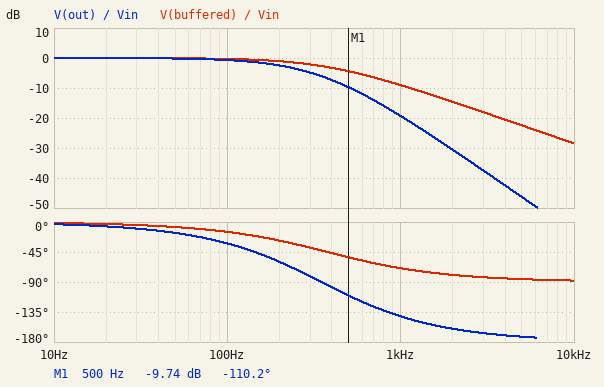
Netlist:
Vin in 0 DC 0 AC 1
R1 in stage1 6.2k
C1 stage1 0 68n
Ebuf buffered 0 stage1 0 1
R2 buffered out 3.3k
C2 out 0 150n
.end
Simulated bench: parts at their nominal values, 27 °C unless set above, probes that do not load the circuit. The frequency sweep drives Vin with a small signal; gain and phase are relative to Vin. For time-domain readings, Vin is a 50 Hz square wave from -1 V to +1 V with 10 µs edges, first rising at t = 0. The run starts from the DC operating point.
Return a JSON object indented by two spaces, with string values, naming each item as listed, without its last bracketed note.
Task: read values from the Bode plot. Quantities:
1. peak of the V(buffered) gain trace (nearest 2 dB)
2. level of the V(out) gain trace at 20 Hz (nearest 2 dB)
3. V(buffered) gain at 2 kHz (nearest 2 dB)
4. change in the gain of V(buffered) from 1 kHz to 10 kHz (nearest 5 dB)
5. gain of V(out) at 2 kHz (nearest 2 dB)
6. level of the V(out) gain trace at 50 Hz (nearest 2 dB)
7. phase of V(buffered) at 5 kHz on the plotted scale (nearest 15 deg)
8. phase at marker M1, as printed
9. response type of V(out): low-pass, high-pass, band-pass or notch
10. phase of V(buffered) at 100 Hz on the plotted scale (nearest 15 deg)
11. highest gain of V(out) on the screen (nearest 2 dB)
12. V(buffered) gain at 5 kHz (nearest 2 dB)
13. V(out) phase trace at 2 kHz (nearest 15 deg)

{
  "peak of the V(buffered) gain trace": "0 dB",
  "level of the V(out) gain trace at 20 Hz": "0 dB",
  "V(buffered) gain at 2 kHz": "-14 dB",
  "change in the gain of V(buffered) from 1 kHz to 10 kHz": "-20 dB",
  "gain of V(out) at 2 kHz": "-30 dB",
  "level of the V(out) gain trace at 50 Hz": "0 dB",
  "phase of V(buffered) at 5 kHz on the plotted scale": "-90 deg",
  "phase at marker M1, as printed": "-110.2 deg",
  "response type of V(out): low-pass, high-pass, band-pass or notch": "low-pass",
  "phase of V(buffered) at 100 Hz on the plotted scale": "-15 deg",
  "highest gain of V(out) on the screen": "0 dB",
  "V(buffered) gain at 5 kHz": "-22 dB",
  "V(out) phase trace at 2 kHz": "-165 deg"
}
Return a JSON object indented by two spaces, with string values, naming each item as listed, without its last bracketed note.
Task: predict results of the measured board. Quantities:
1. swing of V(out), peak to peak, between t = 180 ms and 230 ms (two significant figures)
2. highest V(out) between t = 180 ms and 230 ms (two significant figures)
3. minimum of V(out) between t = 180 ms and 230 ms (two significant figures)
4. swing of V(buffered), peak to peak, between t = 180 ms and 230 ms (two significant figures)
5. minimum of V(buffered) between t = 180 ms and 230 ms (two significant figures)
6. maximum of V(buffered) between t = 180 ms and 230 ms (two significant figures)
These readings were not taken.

{
  "swing of V(out), peak to peak, between t = 180 ms and 230 ms": "2.0 V",
  "highest V(out) between t = 180 ms and 230 ms": "1.0 V",
  "minimum of V(out) between t = 180 ms and 230 ms": "-1.0 V",
  "swing of V(buffered), peak to peak, between t = 180 ms and 230 ms": "2.0 V",
  "minimum of V(buffered) between t = 180 ms and 230 ms": "-1.0 V",
  "maximum of V(buffered) between t = 180 ms and 230 ms": "1.0 V"
}
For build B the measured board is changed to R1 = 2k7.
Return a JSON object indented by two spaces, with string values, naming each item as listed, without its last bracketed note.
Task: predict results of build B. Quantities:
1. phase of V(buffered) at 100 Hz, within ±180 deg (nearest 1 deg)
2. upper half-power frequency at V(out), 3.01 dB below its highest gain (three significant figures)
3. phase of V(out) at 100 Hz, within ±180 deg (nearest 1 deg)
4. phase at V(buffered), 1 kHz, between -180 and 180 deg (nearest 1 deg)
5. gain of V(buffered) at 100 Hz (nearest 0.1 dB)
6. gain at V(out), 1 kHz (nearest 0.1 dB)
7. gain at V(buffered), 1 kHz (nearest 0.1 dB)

{
  "phase of V(buffered) at 100 Hz, within ±180 deg": "-7 deg",
  "upper half-power frequency at V(out), 3.01 dB below its highest gain": "288 Hz",
  "phase of V(out) at 100 Hz, within ±180 deg": "-24 deg",
  "phase at V(buffered), 1 kHz, between -180 and 180 deg": "-49 deg",
  "gain of V(buffered) at 100 Hz": "-0.1 dB",
  "gain at V(out), 1 kHz": "-14.0 dB",
  "gain at V(buffered), 1 kHz": "-3.7 dB"
}
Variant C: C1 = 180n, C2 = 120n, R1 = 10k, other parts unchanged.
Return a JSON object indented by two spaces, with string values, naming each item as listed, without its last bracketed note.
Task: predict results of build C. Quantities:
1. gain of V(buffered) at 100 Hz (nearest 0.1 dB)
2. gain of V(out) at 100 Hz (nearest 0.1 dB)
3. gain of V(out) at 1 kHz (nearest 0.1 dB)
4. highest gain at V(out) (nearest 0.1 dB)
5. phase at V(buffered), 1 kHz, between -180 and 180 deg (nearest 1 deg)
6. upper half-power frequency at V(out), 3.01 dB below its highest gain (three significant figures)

{
  "gain of V(buffered) at 100 Hz": "-3.6 dB",
  "gain of V(out) at 100 Hz": "-3.8 dB",
  "gain of V(out) at 1 kHz": "-29.7 dB",
  "highest gain at V(out)": "0 dB",
  "phase at V(buffered), 1 kHz, between -180 and 180 deg": "-85 deg",
  "upper half-power frequency at V(out), 3.01 dB below its highest gain": "84.6 Hz"
}
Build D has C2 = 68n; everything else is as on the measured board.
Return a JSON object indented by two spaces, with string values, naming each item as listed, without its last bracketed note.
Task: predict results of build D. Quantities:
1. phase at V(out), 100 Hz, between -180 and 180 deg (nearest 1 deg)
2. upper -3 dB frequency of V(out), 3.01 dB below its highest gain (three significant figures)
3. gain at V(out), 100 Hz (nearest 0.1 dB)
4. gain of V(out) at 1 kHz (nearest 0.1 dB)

{
  "phase at V(out), 100 Hz, between -180 and 180 deg": "-23 deg",
  "upper -3 dB frequency of V(out), 3.01 dB below its highest gain": "311 Hz",
  "gain at V(out), 100 Hz": "-0.4 dB",
  "gain of V(out) at 1 kHz": "-13.8 dB"
}
